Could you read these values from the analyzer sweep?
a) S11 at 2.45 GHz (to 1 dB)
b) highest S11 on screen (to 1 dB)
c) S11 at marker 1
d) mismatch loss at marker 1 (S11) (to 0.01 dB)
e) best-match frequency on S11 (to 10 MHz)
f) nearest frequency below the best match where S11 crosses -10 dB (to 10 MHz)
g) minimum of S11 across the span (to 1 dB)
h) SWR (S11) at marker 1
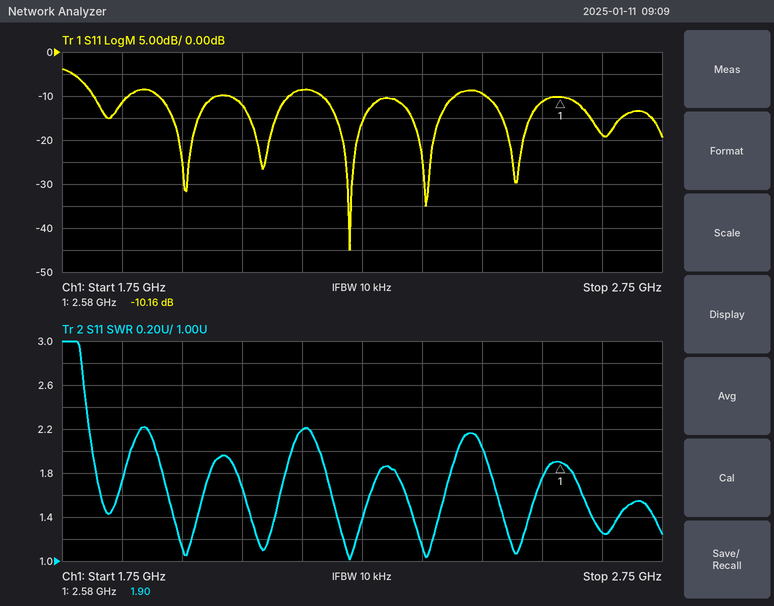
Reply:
-9 dB
-4 dB
-10.16 dB
0.44 dB
2.23 GHz
2.18 GHz
-45 dB
1.90
